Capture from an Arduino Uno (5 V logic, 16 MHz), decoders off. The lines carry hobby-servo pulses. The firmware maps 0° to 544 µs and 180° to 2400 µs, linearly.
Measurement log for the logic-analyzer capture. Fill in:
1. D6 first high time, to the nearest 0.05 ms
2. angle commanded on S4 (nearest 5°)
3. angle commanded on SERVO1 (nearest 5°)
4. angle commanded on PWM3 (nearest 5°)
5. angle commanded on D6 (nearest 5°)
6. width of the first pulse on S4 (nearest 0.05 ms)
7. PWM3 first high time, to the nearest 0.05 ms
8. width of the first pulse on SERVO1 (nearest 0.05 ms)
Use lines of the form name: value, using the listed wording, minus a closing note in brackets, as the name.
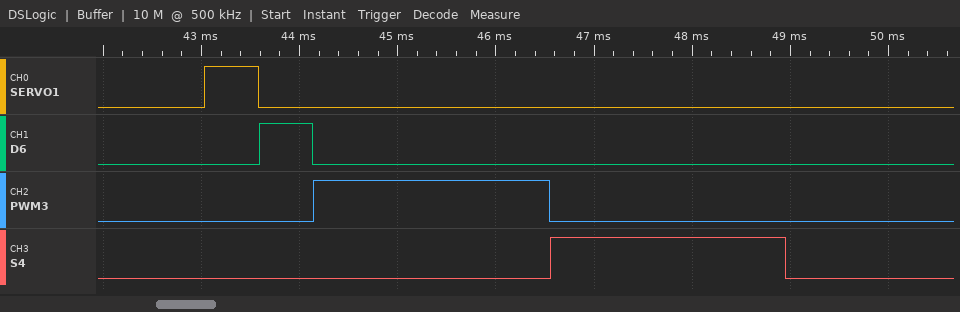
D6 first high time, to the nearest 0.05 ms: 0.55 ms
angle commanded on S4: 180°
angle commanded on SERVO1: 0°
angle commanded on PWM3: 180°
angle commanded on D6: 0°
width of the first pulse on S4: 2.40 ms
PWM3 first high time, to the nearest 0.05 ms: 2.40 ms
width of the first pulse on SERVO1: 0.55 ms
